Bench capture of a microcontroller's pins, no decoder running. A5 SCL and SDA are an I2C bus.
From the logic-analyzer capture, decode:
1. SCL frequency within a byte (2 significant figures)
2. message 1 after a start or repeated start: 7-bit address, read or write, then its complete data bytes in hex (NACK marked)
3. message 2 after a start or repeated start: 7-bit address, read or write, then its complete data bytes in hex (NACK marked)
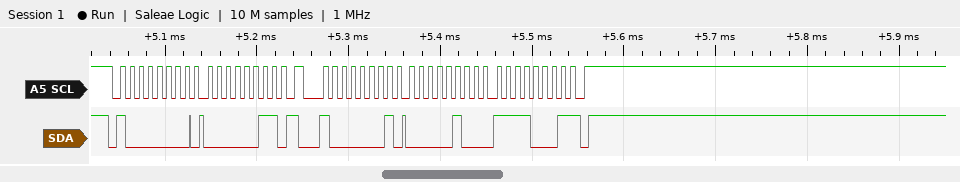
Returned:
100 kHz
0x40 write: 03
0x40 read: 04 F1 NACK
